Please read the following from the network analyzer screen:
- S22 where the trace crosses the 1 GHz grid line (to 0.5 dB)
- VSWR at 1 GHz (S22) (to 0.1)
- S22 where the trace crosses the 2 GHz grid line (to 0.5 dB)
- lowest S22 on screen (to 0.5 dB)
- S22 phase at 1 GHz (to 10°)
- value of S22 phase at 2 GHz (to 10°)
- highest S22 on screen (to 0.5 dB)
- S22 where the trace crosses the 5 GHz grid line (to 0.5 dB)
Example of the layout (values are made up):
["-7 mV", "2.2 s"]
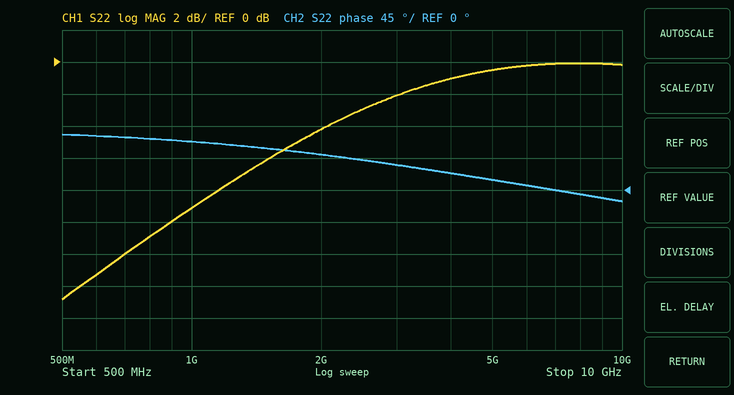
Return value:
["-9.0 dB", "2.1", "-4.0 dB", "-15.0 dB", "70°", "50°", "0.0 dB", "-0.5 dB"]
